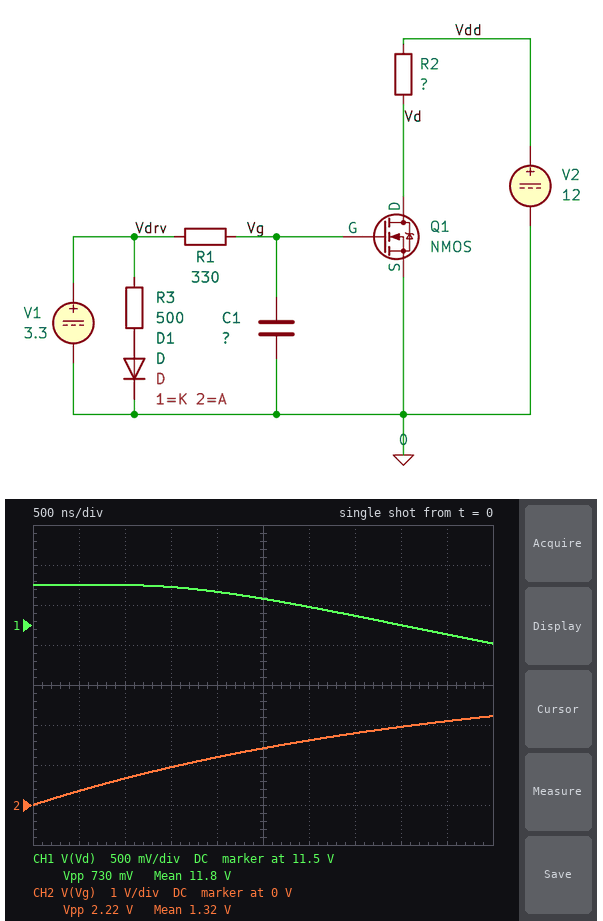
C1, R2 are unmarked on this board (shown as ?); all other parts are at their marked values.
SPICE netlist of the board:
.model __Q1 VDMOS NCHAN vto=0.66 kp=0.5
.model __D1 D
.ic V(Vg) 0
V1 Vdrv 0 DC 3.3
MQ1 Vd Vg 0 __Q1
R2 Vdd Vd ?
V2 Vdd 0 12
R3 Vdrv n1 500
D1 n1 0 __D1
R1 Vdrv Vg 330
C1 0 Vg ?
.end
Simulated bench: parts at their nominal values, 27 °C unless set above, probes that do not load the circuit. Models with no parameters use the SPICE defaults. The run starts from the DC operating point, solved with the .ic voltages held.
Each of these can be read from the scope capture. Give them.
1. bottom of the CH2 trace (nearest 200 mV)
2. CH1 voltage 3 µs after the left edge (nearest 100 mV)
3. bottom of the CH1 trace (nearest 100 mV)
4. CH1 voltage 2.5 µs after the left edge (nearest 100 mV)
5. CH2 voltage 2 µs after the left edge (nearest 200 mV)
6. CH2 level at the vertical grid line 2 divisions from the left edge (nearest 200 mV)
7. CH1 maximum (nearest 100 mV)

0 V
11.7 V
11.3 V
11.8 V
1.2 V
600 mV
12.0 V
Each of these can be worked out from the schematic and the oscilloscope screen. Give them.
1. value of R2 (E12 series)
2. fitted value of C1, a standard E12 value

1.2 Ω
12 nF
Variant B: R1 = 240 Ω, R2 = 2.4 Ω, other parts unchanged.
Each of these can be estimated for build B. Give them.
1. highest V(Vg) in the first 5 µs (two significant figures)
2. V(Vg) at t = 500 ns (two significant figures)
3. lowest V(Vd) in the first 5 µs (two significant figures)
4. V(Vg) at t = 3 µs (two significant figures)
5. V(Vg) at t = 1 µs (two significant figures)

2.6 V
470 mV
9.8 V
2.0 V
880 mV
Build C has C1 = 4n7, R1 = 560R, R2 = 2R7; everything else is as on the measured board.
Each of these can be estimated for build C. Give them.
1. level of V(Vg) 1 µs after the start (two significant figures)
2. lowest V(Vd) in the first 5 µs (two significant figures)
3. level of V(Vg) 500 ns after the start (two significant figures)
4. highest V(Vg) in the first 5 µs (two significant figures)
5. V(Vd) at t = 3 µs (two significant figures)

830 mV
9.7 V
440 mV
2.5 V
11 V
